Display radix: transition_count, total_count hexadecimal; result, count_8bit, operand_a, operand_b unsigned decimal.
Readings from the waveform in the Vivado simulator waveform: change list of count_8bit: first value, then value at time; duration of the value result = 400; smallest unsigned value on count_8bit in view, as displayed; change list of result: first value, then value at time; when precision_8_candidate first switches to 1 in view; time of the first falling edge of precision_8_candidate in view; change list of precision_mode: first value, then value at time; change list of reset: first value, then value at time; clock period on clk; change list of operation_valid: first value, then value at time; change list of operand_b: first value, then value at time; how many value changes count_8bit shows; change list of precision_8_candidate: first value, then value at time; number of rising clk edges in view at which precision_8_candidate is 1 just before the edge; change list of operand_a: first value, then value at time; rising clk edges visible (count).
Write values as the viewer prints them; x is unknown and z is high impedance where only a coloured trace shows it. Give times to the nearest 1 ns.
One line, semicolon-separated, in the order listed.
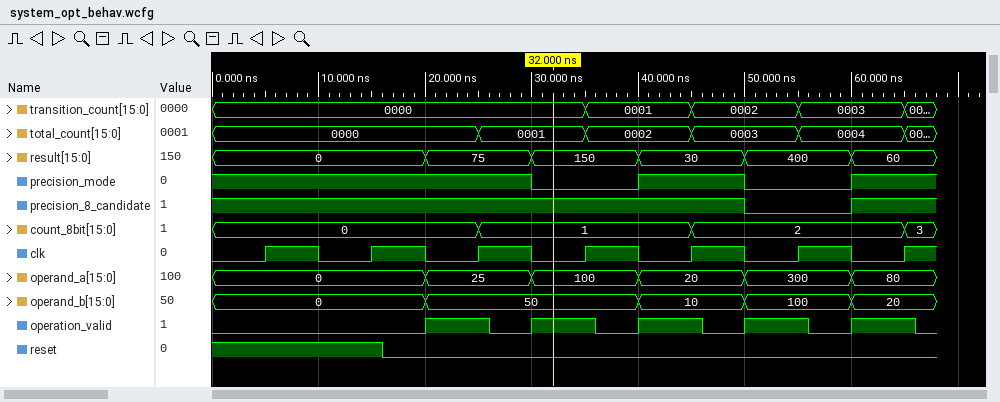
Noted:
0, 1 at 25 ns, 2 at 45 ns, 3 at 65 ns; 10 ns; 0; 0, 75 at 20 ns, 150 at 30 ns, 30 at 40 ns, 400 at 50 ns, 60 at 60 ns; 60 ns; 50 ns; 1, 0 at 30 ns, 1 at 40 ns, 0 at 50 ns, 1 at 60 ns; 1, 0 at 16 ns; 10 ns; 0, 1 at 20 ns, 0 at 26 ns, 1 at 30 ns, 0 at 36 ns, 1 at 40 ns, 0 at 46 ns, 1 at 50 ns, 0 at 56 ns, 1 at 60 ns, 0 at 66 ns; 0, 50 at 20 ns, 10 at 40 ns, 100 at 50 ns, 20 at 60 ns; 3; 1, 0 at 50 ns, 1 at 60 ns; 6; 0, 25 at 20 ns, 100 at 30 ns, 20 at 40 ns, 300 at 50 ns, 80 at 60 ns; 7
